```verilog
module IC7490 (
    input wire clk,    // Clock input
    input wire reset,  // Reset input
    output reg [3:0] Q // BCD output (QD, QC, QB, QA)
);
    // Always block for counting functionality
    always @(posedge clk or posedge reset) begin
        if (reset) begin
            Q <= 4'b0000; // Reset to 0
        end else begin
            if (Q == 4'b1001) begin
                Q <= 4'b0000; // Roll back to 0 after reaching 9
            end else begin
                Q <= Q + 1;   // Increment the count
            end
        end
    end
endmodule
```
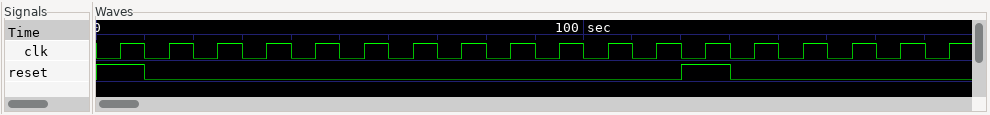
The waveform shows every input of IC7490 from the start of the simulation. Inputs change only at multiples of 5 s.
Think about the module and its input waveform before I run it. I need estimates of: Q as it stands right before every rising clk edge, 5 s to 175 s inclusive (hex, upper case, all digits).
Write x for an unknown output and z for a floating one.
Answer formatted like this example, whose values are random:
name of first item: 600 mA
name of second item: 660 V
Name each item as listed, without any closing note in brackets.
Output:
Q as it stands right before every rising clk edge, 5 s to 175 s inclusive: 0, 0, 1, 2, 3, 4, 5, 6, 7, 8, 9, 0, 0, 0, 1, 2, 3, 4
